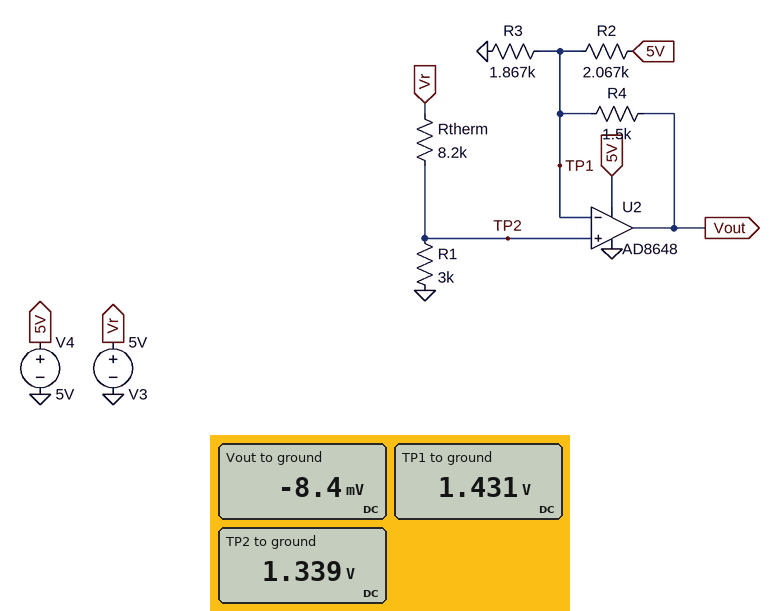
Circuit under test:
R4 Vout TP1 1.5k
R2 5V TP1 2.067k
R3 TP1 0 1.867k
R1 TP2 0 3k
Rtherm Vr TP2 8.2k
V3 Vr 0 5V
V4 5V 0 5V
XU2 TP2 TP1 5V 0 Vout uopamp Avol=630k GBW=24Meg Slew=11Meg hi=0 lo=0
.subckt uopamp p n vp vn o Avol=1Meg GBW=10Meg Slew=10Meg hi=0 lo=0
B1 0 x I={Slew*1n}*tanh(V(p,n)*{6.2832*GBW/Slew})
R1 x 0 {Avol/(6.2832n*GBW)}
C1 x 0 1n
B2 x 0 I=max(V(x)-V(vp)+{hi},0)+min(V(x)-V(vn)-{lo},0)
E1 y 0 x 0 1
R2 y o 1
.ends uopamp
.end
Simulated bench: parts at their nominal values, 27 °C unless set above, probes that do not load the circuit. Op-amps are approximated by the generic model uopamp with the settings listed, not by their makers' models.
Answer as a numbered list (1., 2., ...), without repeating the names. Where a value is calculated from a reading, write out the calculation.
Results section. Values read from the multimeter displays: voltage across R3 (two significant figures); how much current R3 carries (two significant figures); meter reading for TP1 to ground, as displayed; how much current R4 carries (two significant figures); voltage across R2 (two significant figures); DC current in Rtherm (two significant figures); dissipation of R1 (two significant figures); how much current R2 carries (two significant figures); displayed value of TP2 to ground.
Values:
1. 1.431 V = 1.4 V
2. (1.431 V) / 1.867 kΩ = 770 µA
3. 1.431 V
4. (1.431 V - (-8.4 mV)) / 1.5 kΩ = 960 µA
5. 5 V - 1.431 V = 3.6 V
6. (5 V - 1.339 V) / 8.2 kΩ = 450 µA
7. (1.339 V)^2 / 3 kΩ = 600 µW
8. (5 V - 1.431 V) / 2.067 kΩ = 1.7 mA
9. 1.339 V
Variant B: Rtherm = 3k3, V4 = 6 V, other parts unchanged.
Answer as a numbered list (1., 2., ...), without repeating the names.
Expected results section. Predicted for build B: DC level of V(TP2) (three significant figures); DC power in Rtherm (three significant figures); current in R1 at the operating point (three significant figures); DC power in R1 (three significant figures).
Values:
1. 2.38 V
2. 2.08 mW
3. 794 µA
4. 1.89 mW
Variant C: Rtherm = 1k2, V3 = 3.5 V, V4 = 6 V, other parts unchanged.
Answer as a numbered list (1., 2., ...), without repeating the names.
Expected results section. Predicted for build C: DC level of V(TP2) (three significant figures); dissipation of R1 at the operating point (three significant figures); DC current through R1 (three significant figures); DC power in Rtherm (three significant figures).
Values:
1. 2.50 V
2. 2.08 mW
3. 833 µA
4. 833 µW
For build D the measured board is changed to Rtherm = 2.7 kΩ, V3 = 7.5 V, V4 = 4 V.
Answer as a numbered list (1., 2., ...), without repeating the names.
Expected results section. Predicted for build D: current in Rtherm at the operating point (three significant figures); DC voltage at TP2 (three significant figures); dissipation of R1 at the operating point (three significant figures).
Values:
1. 1.32 mA
2. 3.95 V
3. 5.19 mW
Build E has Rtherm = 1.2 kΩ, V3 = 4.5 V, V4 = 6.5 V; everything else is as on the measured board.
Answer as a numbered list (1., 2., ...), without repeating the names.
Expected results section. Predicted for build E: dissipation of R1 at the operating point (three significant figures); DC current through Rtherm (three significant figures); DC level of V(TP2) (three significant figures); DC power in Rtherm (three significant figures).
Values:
1. 3.44 mW
2. 1.07 mA
3. 3.21 V
4. 1.38 mW
